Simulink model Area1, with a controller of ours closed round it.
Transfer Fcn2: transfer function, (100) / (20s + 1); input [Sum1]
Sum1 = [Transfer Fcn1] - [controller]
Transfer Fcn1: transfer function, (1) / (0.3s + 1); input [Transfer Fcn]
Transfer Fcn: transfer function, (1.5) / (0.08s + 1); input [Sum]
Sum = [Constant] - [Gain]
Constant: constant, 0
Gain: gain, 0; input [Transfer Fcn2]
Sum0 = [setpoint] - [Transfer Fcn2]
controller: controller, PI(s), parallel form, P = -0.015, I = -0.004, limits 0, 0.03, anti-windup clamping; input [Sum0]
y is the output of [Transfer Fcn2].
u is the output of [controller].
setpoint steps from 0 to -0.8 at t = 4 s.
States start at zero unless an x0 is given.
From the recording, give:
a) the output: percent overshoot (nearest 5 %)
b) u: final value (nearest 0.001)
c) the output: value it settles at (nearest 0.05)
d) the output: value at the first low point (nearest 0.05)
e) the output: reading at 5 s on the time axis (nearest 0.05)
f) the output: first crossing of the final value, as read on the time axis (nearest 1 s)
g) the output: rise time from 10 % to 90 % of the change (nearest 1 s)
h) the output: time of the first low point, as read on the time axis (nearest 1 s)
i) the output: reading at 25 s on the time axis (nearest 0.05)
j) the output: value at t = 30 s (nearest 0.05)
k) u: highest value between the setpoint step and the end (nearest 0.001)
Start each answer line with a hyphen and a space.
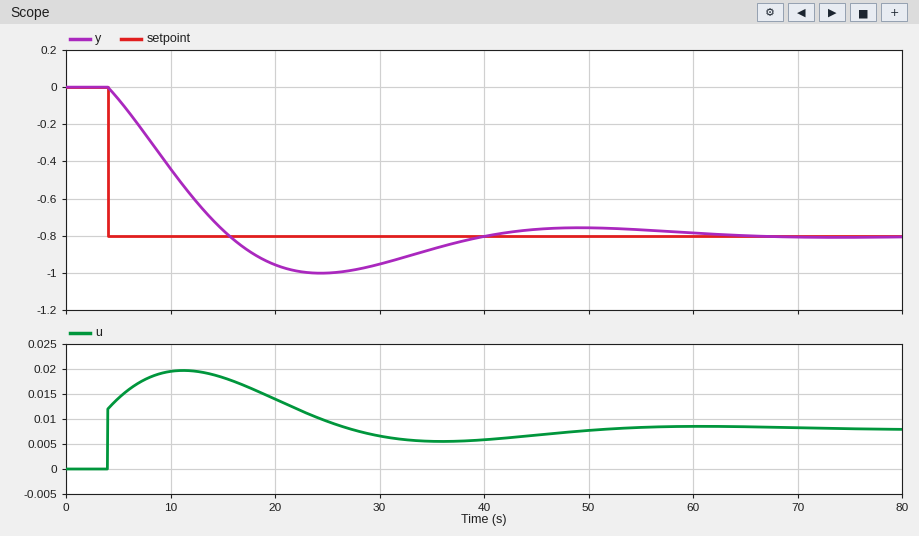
- 25 %
- 0.008
- -0.80
- -1.00
- -0.05
- 16 s
- 9 s
- 24 s
- -1.00
- -0.95
- 0.020
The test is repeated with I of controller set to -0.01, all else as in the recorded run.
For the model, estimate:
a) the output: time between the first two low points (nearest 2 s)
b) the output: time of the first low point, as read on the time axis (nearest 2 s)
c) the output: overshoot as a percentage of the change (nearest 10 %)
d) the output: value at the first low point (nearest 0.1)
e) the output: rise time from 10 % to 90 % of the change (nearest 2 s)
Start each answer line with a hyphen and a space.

- 30 s
- 18 s
- 40 %
- -1.1
- 6 s
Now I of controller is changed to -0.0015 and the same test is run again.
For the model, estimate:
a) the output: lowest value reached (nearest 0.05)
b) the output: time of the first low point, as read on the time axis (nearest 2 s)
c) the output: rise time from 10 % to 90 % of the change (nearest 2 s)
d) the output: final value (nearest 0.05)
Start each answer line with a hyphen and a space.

- -0.85
- 40 s
- 16 s
- -0.80
